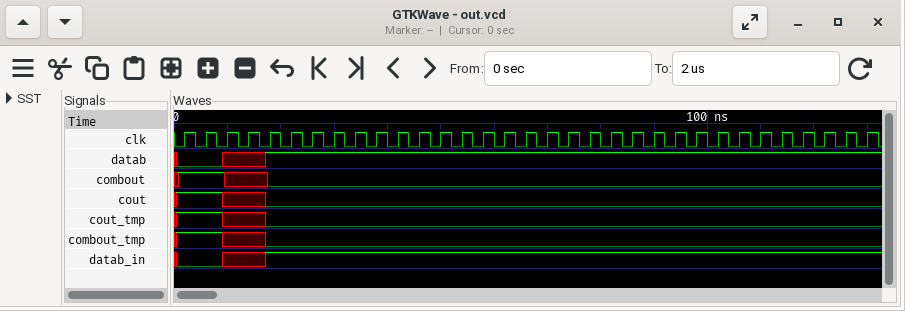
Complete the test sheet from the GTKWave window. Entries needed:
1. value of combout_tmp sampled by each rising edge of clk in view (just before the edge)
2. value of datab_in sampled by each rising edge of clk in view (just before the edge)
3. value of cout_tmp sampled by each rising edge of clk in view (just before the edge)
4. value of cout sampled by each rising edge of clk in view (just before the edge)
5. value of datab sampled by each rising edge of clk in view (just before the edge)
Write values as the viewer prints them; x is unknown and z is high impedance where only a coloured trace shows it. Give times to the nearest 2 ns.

1 1 x x 0 0 0 0 0 0 0 0 0 0 0 0 0 0 0 0 0 0 0 0 0 0 0 0 0 0 0 0 0
0 0 x x 1 1 1 1 1 1 1 1 1 1 1 1 1 1 1 1 1 1 1 1 1 1 1 1 1 1 1 1 1
1 1 x x 0 0 0 0 0 0 0 0 0 0 0 0 0 0 0 0 0 0 0 0 0 0 0 0 0 0 0 0 0
1 1 x x 0 0 0 0 0 0 0 0 0 0 0 0 0 0 0 0 0 0 0 0 0 0 0 0 0 0 0 0 0
0 0 x x 1 1 1 1 1 1 1 1 1 1 1 1 1 1 1 1 1 1 1 1 1 1 1 1 1 1 1 1 1
